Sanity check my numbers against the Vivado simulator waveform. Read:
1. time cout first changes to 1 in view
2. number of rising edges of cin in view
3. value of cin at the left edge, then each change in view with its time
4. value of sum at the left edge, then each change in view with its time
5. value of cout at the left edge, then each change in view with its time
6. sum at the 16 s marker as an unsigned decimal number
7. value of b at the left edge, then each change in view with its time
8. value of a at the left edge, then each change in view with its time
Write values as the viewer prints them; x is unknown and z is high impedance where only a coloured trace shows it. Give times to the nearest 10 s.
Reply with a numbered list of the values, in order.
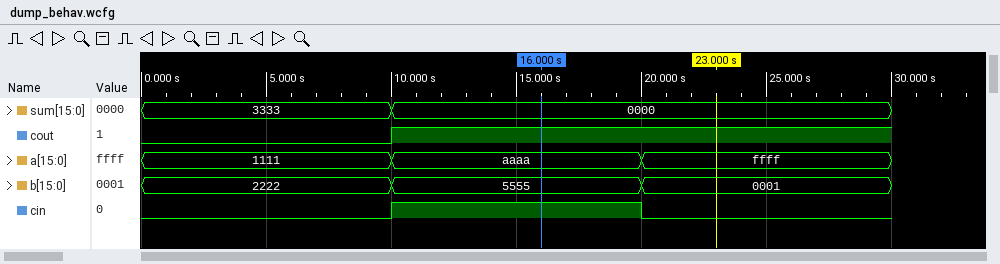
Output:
1. 10 s
2. 1
3. 0, 1 at 10 s, 0 at 20 s
4. 3333, 0000 at 10 s
5. 0, 1 at 10 s
6. 0
7. 2222, 5555 at 10 s, 0001 at 20 s
8. 1111, aaaa at 10 s, ffff at 20 s
